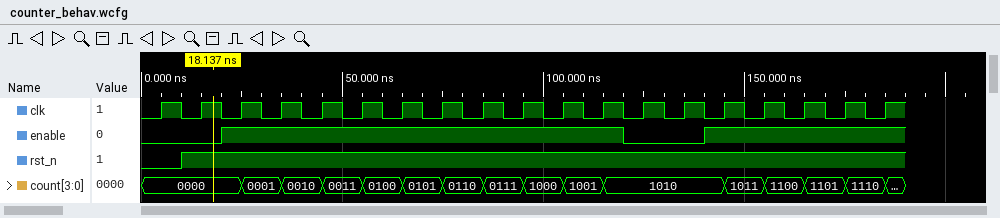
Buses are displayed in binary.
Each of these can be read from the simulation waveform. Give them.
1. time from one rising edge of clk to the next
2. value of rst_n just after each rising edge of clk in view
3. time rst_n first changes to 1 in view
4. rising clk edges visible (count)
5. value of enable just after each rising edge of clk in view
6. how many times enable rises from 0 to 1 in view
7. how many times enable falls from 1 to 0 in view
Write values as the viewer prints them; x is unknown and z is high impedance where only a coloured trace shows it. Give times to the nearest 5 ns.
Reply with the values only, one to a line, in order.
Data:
10 ns
0 1 1 1 1 1 1 1 1 1 1 1 1 1 1 1 1 1 1
10 ns
19
0 0 1 1 1 1 1 1 1 1 1 1 0 0 1 1 1 1 1
2
1
